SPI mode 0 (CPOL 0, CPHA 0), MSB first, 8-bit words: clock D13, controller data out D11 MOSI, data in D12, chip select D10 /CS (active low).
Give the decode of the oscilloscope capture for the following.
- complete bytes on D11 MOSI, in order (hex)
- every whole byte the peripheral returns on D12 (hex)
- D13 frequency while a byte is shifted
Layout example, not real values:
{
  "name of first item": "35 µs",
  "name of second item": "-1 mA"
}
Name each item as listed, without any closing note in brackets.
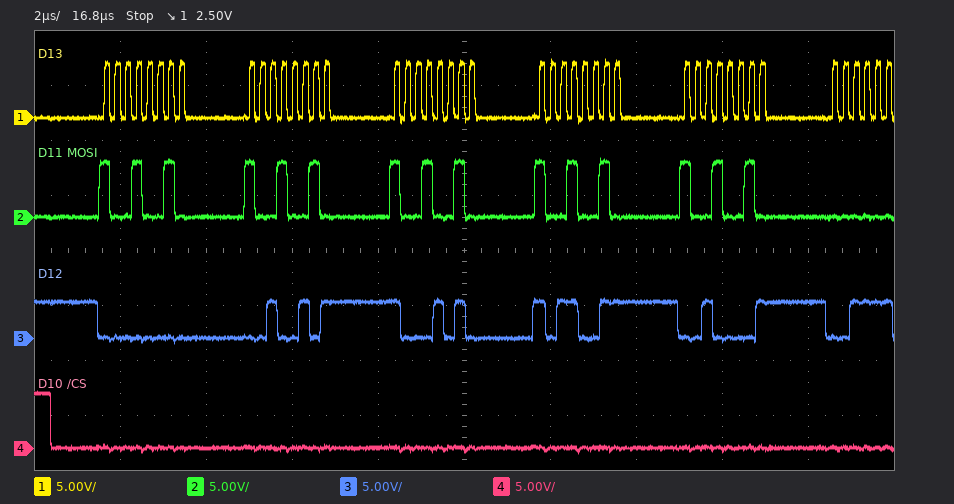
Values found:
{
  "complete bytes on D11 MOSI, in order": "92 92 92 92 92",
  "every whole byte the peripheral returns on D12": "00 25 8A B3 21",
  "D13 frequency while a byte is shifted": "4 MHz"
}
